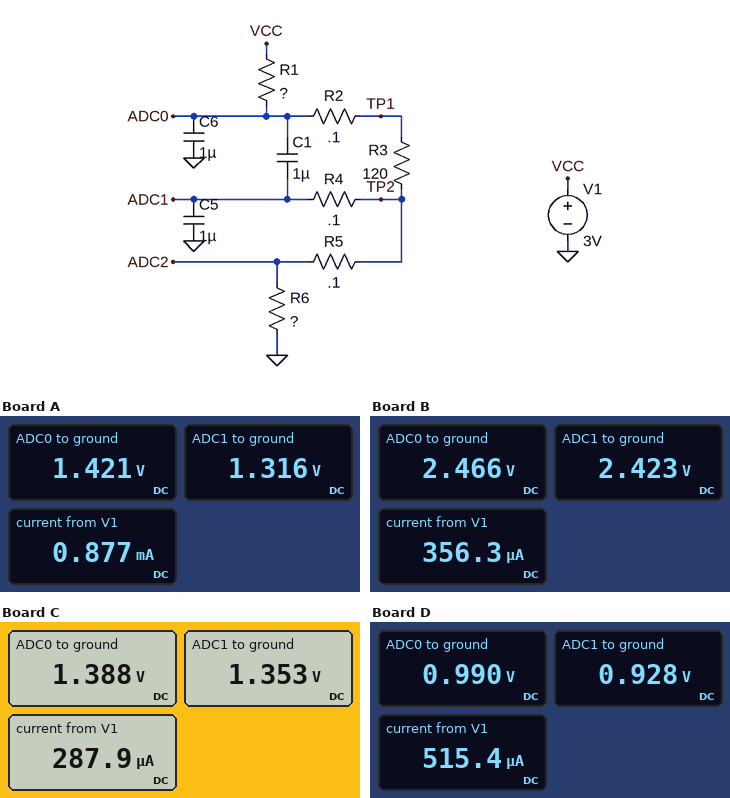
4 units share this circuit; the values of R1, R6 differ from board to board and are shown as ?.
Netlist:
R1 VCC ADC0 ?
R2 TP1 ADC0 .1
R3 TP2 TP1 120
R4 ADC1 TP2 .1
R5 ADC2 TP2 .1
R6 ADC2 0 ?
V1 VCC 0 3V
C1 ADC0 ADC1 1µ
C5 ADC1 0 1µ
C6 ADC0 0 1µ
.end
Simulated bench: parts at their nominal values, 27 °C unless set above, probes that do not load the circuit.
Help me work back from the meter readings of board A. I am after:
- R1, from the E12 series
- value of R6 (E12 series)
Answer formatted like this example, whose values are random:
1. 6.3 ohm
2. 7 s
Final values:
1. 1.8 kΩ
2. 1.5 kΩ
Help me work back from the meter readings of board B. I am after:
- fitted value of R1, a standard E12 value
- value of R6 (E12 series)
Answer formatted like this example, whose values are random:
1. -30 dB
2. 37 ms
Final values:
1. 1.5 kΩ
2. 6.8 kΩ
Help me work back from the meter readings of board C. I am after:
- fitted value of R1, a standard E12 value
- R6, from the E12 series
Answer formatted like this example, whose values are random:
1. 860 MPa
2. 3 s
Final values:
1. 5.6 kΩ
2. 4.7 kΩ
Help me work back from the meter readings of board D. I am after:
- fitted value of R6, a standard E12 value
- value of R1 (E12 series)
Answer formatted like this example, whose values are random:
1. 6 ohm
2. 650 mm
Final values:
1. 1.8 kΩ
2. 3.9 kΩ
